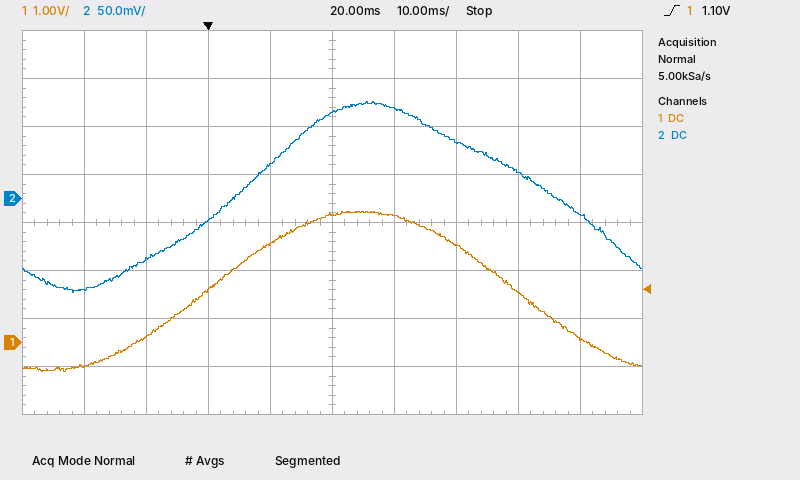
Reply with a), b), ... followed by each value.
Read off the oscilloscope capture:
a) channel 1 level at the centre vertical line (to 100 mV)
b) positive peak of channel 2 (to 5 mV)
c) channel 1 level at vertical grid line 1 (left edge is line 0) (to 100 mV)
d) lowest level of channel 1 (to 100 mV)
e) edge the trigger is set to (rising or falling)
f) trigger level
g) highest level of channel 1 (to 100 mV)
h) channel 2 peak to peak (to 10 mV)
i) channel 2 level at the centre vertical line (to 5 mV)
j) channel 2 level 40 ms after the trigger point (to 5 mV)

a) 2.7 V
b) 100 mV
c) -500 mV
d) -600 mV
e) rising
f) 1.10 V
g) 2.7 V
h) 200 mV
i) 90 mV
j) 60 mV
